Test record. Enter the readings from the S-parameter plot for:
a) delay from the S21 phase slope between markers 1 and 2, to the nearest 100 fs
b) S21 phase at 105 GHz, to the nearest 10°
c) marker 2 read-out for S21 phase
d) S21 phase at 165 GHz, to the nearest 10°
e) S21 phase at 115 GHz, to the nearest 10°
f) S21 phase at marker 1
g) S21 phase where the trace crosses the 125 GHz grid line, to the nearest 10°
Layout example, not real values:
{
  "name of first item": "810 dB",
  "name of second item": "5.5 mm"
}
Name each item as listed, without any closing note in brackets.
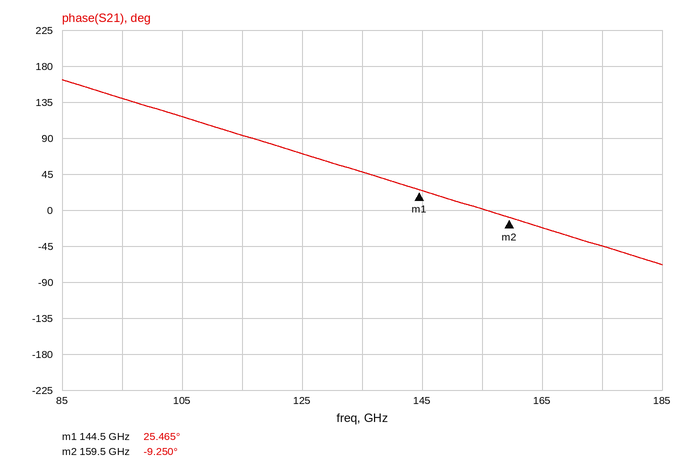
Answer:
{
  "delay from the S21 phase slope between markers 1 and 2, to the nearest 100 fs": "6.4 ps",
  "S21 phase at 105 GHz, to the nearest 10°": "120°",
  "marker 2 read-out for S21 phase": "-9.250°",
  "S21 phase at 165 GHz, to the nearest 10°": "-20°",
  "S21 phase at 115 GHz, to the nearest 10°": "90°",
  "S21 phase at marker 1": "25.465°",
  "S21 phase where the trace crosses the 125 GHz grid line, to the nearest 10°": "70°"
}
